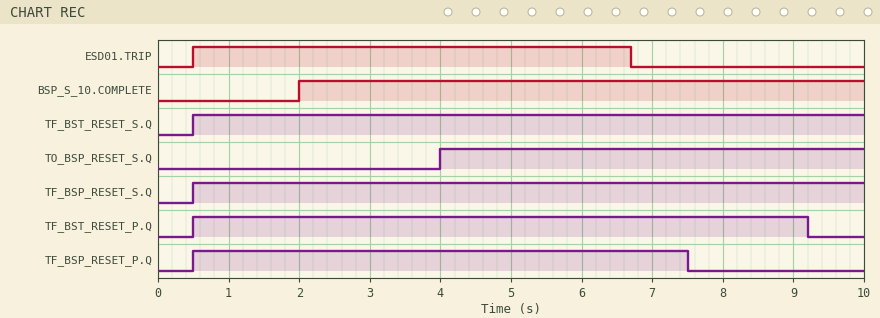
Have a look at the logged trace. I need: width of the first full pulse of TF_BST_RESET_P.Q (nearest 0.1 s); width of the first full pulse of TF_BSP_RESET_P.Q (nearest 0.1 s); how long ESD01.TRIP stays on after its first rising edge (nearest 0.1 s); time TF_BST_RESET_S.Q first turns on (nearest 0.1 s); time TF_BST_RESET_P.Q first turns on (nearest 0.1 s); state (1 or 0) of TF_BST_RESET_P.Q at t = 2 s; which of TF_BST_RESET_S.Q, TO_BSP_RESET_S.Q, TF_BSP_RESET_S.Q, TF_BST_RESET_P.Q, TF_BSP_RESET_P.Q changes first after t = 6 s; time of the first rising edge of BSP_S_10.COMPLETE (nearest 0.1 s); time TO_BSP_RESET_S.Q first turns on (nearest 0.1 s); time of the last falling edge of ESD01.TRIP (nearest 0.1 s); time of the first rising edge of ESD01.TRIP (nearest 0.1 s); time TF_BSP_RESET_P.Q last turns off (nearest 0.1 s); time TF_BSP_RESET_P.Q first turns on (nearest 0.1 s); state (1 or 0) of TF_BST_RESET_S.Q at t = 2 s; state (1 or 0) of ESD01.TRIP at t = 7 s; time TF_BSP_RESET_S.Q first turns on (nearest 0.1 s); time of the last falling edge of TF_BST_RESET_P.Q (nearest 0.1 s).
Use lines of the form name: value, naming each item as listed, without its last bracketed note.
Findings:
width of the first full pulse of TF_BST_RESET_P.Q: 8.7 s
width of the first full pulse of TF_BSP_RESET_P.Q: 7.0 s
how long ESD01.TRIP stays on after its first rising edge: 6.2 s
time TF_BST_RESET_S.Q first turns on: 0.5 s
time TF_BST_RESET_P.Q first turns on: 0.5 s
state (1 or 0) of TF_BST_RESET_P.Q at t = 2 s: 1
which of TF_BST_RESET_S.Q, TO_BSP_RESET_S.Q, TF_BSP_RESET_S.Q, TF_BST_RESET_P.Q, TF_BSP_RESET_P.Q changes first after t = 6 s: TF_BSP_RESET_P.Q
time of the first rising edge of BSP_S_10.COMPLETE: 2.0 s
time TO_BSP_RESET_S.Q first turns on: 4.0 s
time of the last falling edge of ESD01.TRIP: 6.7 s
time of the first rising edge of ESD01.TRIP: 0.5 s
time TF_BSP_RESET_P.Q last turns off: 7.5 s
time TF_BSP_RESET_P.Q first turns on: 0.5 s
state (1 or 0) of TF_BST_RESET_S.Q at t = 2 s: 1
state (1 or 0) of ESD01.TRIP at t = 7 s: 0
time TF_BSP_RESET_S.Q first turns on: 0.5 s
time of the last falling edge of TF_BST_RESET_P.Q: 9.2 s
